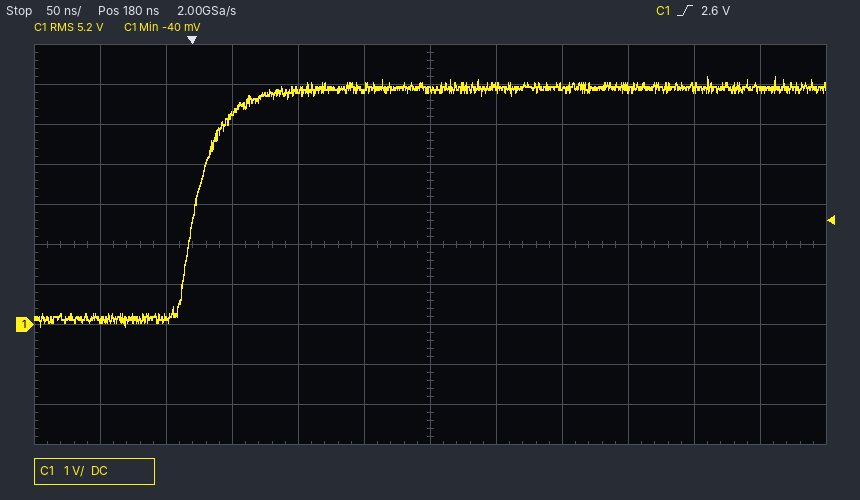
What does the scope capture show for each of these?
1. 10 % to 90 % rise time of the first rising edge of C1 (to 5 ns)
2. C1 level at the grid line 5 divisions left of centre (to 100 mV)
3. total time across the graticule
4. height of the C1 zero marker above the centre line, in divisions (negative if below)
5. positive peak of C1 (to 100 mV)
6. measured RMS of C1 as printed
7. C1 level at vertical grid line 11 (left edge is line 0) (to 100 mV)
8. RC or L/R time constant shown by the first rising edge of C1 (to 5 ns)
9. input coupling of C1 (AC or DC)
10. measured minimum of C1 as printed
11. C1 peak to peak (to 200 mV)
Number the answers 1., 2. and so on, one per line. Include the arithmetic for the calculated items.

1. 40 ns
2. 100 mV
3. 600 ns
4. -2.0 div
5. 6.2 V
6. 5.2 V
7. 5.9 V
8. 40 ns / 2.2 ≈ 18.2 ns, so 20 ns to the nearest 5 ns
9. DC
10. -40 mV
11. 6.2 V
